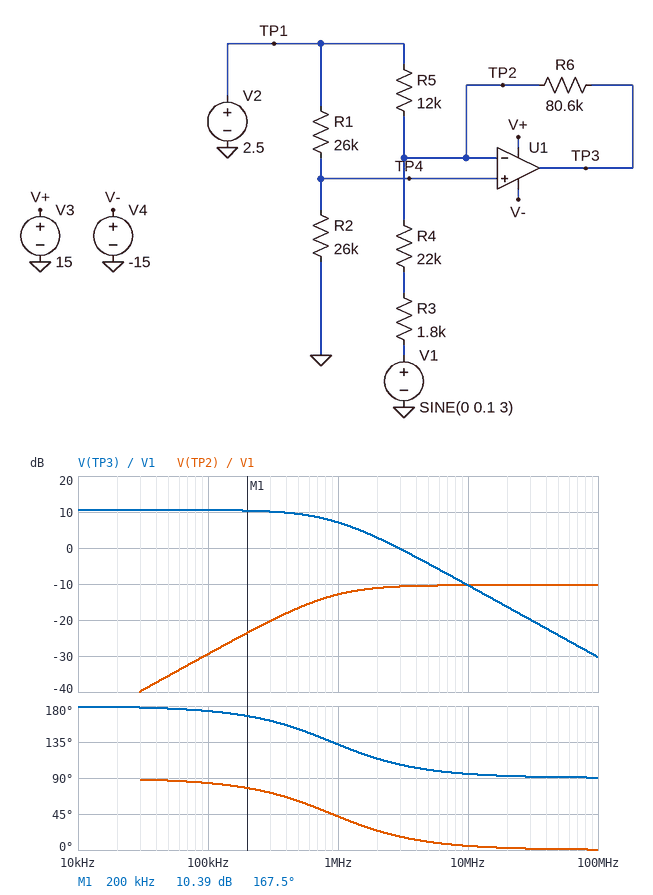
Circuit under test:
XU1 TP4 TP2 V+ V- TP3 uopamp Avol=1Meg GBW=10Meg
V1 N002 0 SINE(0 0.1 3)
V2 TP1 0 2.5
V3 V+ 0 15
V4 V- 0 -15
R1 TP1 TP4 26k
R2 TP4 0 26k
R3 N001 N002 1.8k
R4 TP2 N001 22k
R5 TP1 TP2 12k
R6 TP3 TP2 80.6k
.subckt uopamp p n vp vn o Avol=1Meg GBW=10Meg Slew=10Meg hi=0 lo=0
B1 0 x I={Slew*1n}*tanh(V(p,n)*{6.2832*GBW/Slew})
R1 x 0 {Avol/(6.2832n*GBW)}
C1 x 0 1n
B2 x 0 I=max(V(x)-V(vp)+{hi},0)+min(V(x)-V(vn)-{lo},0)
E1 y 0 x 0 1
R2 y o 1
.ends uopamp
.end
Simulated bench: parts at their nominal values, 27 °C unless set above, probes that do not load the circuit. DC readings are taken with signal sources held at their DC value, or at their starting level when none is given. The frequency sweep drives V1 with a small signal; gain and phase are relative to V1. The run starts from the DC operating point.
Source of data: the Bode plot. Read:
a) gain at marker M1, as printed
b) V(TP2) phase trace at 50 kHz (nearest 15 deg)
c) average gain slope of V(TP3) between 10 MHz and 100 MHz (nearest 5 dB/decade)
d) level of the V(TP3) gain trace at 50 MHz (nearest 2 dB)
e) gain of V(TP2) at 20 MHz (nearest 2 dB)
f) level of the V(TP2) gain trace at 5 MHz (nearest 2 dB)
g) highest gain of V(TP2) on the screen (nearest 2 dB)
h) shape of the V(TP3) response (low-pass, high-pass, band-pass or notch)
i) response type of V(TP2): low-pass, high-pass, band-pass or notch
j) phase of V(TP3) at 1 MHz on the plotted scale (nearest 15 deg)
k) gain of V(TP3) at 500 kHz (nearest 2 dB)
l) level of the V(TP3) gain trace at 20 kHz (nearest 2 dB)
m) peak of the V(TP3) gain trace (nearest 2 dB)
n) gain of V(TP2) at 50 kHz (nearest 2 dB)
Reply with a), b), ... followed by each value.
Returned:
a) 10.39 dB
b) 90 deg
c) -20 dB/decade
d) -24 dB
e) -10 dB
f) -10 dB
g) -10 dB
h) low-pass
i) high-pass
j) 135 deg
k) 10 dB
l) 10 dB
m) 10 dB
n) -36 dB
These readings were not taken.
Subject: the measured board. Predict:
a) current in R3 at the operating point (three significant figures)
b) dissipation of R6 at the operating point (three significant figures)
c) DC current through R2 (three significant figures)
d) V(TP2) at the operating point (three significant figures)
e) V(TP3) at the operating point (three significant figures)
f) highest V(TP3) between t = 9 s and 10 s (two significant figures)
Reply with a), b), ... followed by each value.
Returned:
a) 52.5 µA
b) 215 µW
c) 48.1 µA
d) 1.25 V
e) -2.91 V
f) -2.6 V
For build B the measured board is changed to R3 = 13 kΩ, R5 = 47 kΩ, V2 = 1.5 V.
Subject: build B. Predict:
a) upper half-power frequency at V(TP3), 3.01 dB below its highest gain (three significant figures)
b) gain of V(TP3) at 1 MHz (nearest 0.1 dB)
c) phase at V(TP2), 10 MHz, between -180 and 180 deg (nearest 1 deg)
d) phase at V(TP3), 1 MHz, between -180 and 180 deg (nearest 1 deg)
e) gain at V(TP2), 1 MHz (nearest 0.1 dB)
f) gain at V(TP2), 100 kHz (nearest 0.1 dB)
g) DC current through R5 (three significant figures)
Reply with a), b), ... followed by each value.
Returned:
a) 1.99 MHz
b) 6.3 dB
c) 11 deg
d) 153 deg
e) -13.7 dB
f) -32.8 dB
g) 16.0 µA
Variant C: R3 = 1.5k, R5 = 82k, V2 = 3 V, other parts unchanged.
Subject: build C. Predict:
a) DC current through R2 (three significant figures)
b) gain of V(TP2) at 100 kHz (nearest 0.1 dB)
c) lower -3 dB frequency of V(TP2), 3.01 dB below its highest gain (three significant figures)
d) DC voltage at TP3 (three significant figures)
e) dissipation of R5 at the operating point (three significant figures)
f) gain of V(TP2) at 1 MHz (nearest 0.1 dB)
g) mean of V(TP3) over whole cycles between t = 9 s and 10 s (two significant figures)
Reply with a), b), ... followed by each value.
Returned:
a) 57.7 µA
b) -29.3 dB
c) 1.85 MHz
d) 5.17 V
e) 27.4 µW
f) -10.4 dB
g) 5.2 V
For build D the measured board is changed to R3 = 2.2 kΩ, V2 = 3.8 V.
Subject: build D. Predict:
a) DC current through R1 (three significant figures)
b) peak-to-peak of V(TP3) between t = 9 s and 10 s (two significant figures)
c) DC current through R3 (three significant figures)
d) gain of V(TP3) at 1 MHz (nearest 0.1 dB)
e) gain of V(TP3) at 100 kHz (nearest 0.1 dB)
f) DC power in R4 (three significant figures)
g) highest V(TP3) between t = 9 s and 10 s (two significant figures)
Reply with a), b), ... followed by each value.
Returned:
a) 73.1 µA
b) 670 mV
c) 78.5 µA
d) 7.0 dB
e) 10.4 dB
f) 136 µW
g) -4.2 V
